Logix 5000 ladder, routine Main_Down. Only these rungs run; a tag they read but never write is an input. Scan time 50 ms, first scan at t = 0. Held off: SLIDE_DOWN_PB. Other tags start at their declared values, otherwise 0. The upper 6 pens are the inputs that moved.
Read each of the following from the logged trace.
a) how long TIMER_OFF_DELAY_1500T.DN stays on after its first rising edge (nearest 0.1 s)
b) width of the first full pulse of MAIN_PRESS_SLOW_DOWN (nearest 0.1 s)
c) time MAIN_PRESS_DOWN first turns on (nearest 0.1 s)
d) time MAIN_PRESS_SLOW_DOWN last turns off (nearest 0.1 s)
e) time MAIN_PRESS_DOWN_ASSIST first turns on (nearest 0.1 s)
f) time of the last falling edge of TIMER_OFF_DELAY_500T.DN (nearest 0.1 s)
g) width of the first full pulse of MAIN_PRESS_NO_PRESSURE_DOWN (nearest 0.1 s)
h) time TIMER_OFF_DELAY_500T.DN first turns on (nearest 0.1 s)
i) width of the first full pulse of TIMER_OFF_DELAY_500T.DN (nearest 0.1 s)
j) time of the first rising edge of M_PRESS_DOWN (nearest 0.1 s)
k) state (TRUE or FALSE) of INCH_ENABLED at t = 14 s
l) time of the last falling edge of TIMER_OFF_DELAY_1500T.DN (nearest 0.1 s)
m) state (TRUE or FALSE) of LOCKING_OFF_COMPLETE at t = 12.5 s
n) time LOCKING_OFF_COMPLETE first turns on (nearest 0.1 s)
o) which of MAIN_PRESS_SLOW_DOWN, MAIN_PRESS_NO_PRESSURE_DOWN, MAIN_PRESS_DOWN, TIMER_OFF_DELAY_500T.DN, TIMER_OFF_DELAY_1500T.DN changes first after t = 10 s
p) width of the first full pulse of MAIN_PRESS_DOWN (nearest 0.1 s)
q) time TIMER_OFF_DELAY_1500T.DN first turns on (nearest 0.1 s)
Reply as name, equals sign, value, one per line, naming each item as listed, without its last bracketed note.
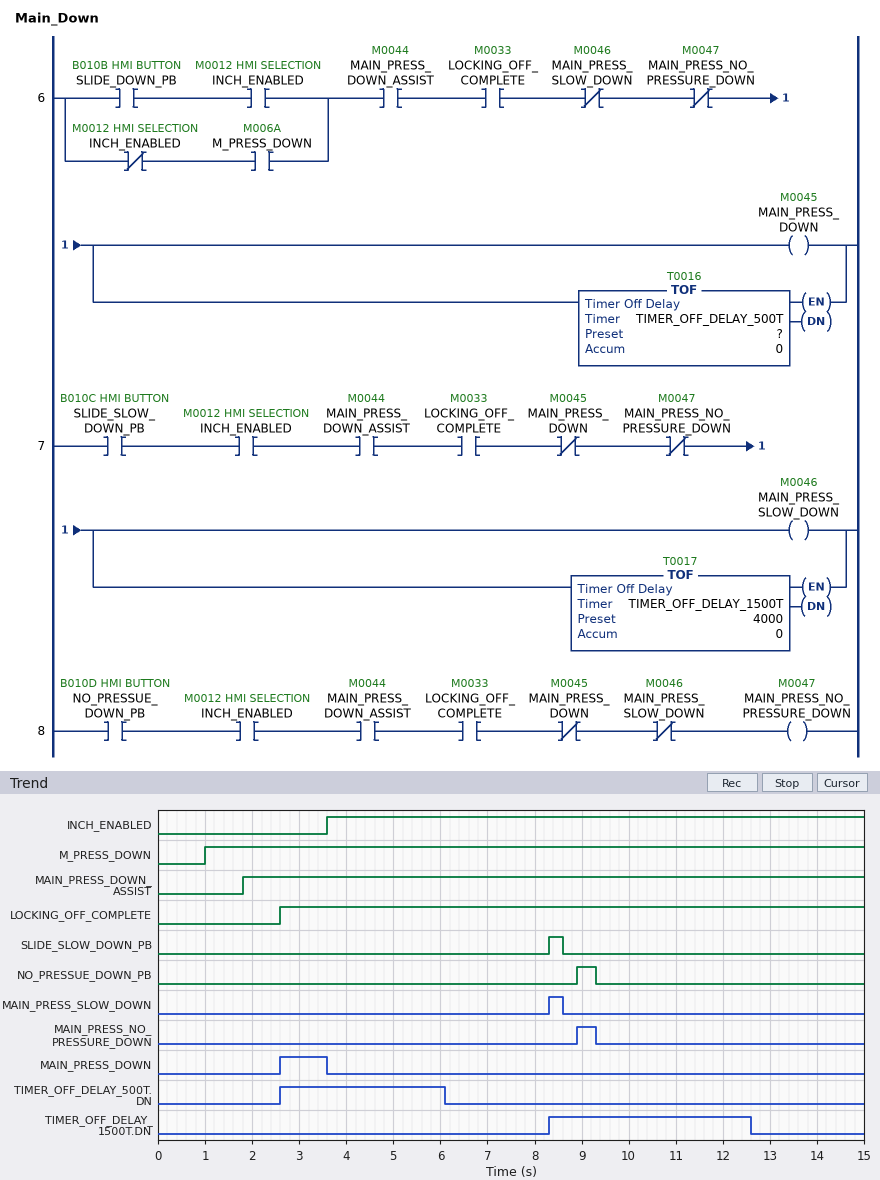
how long TIMER_OFF_DELAY_1500T.DN stays on after its first rising edge = 4.3 s
width of the first full pulse of MAIN_PRESS_SLOW_DOWN = 0.3 s
time MAIN_PRESS_DOWN first turns on = 2.6 s
time MAIN_PRESS_SLOW_DOWN last turns off = 8.6 s
time MAIN_PRESS_DOWN_ASSIST first turns on = 1.8 s
time of the last falling edge of TIMER_OFF_DELAY_500T.DN = 6.1 s
width of the first full pulse of MAIN_PRESS_NO_PRESSURE_DOWN = 0.4 s
time TIMER_OFF_DELAY_500T.DN first turns on = 2.6 s
width of the first full pulse of TIMER_OFF_DELAY_500T.DN = 3.5 s
time of the first rising edge of M_PRESS_DOWN = 1.0 s
state (TRUE or FALSE) of INCH_ENABLED at t = 14 s = TRUE
time of the last falling edge of TIMER_OFF_DELAY_1500T.DN = 12.6 s
state (TRUE or FALSE) of LOCKING_OFF_COMPLETE at t = 12.5 s = TRUE
time LOCKING_OFF_COMPLETE first turns on = 2.6 s
which of MAIN_PRESS_SLOW_DOWN, MAIN_PRESS_NO_PRESSURE_DOWN, MAIN_PRESS_DOWN, TIMER_OFF_DELAY_500T.DN, TIMER_OFF_DELAY_1500T.DN changes first after t = 10 s = TIMER_OFF_DELAY_1500T.DN
width of the first full pulse of MAIN_PRESS_DOWN = 1.0 s
time TIMER_OFF_DELAY_1500T.DN first turns on = 8.3 s
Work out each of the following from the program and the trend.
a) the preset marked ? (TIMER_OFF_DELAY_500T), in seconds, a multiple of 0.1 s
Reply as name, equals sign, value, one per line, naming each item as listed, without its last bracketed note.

the preset marked ? (TIMER_OFF_DELAY_500T), in seconds, a multiple of 0.1 s = 2.5 s
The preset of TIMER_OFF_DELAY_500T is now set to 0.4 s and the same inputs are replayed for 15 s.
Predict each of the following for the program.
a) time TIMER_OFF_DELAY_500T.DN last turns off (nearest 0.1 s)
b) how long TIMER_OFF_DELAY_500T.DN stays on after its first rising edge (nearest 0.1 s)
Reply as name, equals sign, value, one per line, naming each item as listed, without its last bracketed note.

time TIMER_OFF_DELAY_500T.DN last turns off = 4.0 s
how long TIMER_OFF_DELAY_500T.DN stays on after its first rising edge = 1.4 s
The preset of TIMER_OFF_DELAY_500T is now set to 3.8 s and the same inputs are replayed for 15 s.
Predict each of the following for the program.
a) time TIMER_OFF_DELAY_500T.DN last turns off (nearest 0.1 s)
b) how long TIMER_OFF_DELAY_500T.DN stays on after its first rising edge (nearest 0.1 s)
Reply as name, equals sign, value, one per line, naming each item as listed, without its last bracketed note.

time TIMER_OFF_DELAY_500T.DN last turns off = 7.4 s
how long TIMER_OFF_DELAY_500T.DN stays on after its first rising edge = 4.8 s
